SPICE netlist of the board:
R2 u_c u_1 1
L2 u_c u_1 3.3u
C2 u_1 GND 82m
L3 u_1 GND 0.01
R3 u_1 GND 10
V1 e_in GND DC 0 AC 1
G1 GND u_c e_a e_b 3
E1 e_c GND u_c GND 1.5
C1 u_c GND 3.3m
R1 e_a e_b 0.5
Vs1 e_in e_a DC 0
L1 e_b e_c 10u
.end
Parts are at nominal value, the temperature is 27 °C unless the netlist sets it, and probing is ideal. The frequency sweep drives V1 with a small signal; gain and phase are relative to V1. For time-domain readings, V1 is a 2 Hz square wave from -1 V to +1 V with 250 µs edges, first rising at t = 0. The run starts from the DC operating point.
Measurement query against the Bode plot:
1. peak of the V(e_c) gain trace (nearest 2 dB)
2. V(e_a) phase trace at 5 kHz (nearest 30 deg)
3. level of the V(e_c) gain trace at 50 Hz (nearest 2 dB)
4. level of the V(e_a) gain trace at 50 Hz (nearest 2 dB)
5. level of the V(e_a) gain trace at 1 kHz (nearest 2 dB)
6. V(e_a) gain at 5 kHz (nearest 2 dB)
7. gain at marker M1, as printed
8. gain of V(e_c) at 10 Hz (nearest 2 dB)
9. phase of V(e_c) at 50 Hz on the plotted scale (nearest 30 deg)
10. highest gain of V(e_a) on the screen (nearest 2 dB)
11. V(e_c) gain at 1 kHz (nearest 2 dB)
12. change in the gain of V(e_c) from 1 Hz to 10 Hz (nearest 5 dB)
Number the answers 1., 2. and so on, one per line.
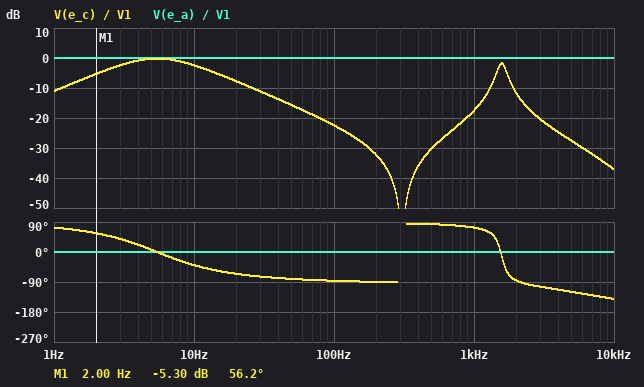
1. 0 dB
2. 0 deg
3. -16 dB
4. 0 dB
5. 0 dB
6. 0 dB
7. -5.30 dB
8. -2 dB
9. -90 deg
10. 0 dB
11. -18 dB
12. 10 dB
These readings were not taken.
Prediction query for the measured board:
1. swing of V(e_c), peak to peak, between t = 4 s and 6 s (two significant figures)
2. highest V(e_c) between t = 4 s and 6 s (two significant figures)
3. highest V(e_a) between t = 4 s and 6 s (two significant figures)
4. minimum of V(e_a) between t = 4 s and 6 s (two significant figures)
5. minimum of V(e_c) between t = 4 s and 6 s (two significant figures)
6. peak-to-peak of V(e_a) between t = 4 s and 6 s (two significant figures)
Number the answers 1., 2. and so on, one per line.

1. 2.6 V
2. 1.3 V
3. 1.0 V
4. -1.0 V
5. -1.3 V
6. 2.0 V
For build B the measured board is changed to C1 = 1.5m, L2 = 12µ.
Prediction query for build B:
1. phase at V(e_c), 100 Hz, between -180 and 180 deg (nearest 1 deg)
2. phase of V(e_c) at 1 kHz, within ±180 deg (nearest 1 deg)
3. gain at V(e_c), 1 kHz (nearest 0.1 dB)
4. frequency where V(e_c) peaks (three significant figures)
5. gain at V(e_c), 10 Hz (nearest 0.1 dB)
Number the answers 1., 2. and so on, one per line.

1. -87 deg
2. 34 deg
3. -4.2 dB
4. 5.51 Hz
5. -2.3 dB
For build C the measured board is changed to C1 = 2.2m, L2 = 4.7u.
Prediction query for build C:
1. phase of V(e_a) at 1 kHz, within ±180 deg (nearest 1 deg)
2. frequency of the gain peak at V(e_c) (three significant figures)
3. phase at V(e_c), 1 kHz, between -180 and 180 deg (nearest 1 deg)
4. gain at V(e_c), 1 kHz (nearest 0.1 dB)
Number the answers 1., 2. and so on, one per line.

1. 0 deg
2. 5.49 Hz
3. 69 deg
4. -14.5 dB
